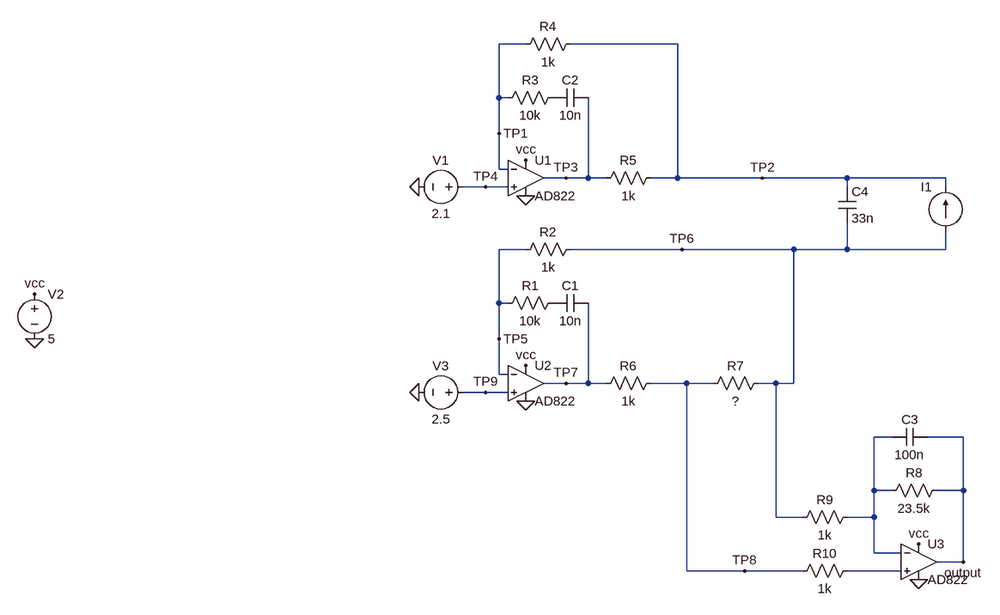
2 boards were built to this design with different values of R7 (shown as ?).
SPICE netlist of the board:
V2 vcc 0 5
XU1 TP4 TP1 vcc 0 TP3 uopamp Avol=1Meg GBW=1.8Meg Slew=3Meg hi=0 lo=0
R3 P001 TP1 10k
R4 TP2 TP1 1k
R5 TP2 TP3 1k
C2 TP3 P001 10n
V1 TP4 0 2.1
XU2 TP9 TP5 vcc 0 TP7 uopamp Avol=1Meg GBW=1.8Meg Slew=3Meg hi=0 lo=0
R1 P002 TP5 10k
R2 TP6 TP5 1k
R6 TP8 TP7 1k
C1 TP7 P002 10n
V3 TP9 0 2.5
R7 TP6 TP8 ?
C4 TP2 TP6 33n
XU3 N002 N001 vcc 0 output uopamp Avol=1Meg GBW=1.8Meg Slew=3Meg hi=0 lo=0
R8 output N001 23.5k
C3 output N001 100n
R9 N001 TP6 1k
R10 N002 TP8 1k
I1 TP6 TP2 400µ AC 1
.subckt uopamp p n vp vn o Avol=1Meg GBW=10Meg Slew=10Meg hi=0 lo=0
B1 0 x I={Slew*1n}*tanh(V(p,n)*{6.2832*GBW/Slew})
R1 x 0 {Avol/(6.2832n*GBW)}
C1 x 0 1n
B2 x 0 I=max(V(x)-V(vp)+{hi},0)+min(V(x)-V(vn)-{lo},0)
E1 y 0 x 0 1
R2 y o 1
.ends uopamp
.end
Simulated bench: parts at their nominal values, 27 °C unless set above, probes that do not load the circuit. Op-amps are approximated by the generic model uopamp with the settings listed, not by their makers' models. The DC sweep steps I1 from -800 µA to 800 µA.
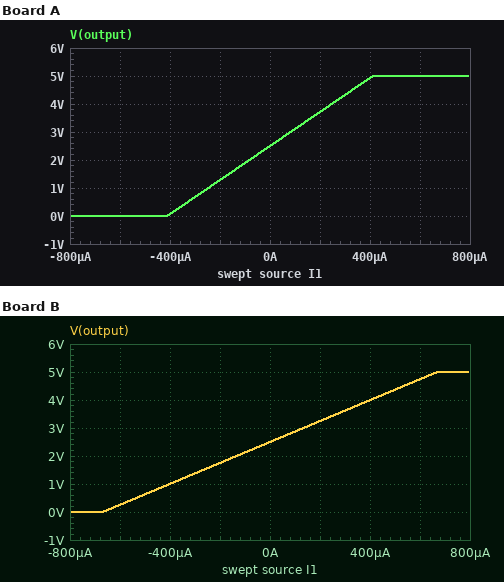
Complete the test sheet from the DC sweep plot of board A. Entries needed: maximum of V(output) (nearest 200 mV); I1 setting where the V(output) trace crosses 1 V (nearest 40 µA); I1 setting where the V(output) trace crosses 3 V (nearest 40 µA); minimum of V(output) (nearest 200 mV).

5.0 V
-240 µA
80 µA
0 V
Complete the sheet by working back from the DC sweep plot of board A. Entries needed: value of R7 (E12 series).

330 Ω
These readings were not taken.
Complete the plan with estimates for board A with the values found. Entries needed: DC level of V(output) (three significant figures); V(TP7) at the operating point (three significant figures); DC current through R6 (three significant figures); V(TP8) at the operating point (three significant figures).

4.93 V
2.90 V
301 µA
2.60 V
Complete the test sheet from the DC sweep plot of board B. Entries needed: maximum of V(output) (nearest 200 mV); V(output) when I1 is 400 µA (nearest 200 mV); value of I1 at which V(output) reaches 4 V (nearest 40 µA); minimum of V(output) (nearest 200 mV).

5.0 V
4.0 V
400 µA
0 V
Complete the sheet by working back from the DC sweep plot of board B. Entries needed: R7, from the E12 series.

180 Ω
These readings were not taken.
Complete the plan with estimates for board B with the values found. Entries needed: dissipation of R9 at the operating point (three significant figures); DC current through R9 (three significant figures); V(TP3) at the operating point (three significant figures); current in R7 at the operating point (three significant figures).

3.72 µW
61.0 µA
1.70 V
339 µA
